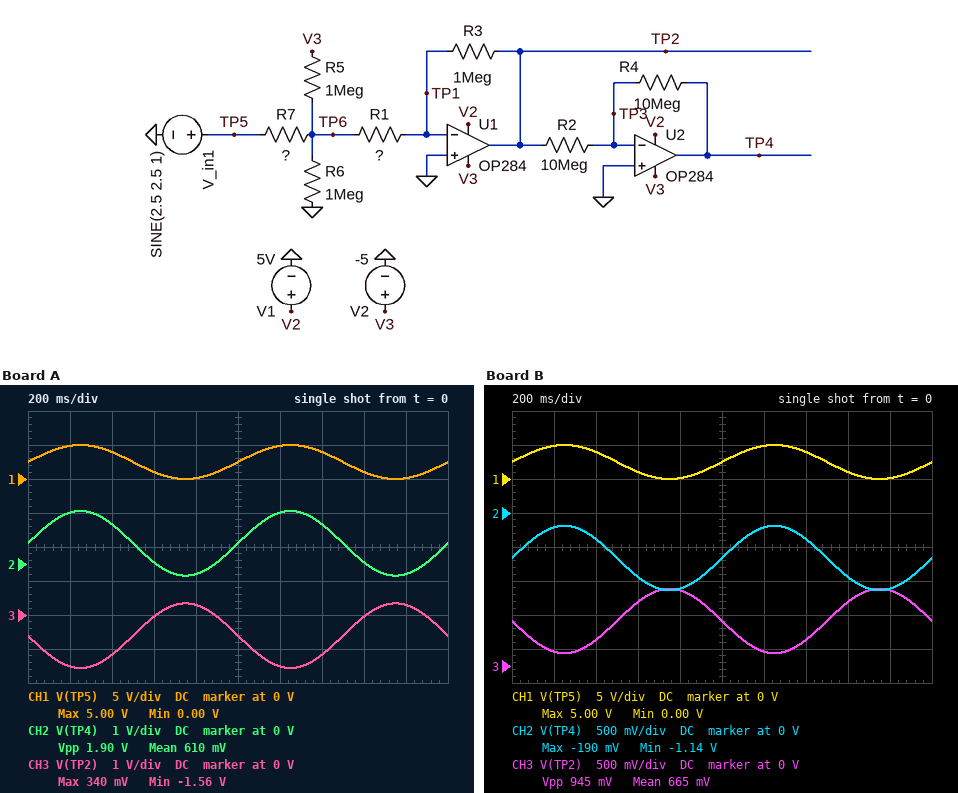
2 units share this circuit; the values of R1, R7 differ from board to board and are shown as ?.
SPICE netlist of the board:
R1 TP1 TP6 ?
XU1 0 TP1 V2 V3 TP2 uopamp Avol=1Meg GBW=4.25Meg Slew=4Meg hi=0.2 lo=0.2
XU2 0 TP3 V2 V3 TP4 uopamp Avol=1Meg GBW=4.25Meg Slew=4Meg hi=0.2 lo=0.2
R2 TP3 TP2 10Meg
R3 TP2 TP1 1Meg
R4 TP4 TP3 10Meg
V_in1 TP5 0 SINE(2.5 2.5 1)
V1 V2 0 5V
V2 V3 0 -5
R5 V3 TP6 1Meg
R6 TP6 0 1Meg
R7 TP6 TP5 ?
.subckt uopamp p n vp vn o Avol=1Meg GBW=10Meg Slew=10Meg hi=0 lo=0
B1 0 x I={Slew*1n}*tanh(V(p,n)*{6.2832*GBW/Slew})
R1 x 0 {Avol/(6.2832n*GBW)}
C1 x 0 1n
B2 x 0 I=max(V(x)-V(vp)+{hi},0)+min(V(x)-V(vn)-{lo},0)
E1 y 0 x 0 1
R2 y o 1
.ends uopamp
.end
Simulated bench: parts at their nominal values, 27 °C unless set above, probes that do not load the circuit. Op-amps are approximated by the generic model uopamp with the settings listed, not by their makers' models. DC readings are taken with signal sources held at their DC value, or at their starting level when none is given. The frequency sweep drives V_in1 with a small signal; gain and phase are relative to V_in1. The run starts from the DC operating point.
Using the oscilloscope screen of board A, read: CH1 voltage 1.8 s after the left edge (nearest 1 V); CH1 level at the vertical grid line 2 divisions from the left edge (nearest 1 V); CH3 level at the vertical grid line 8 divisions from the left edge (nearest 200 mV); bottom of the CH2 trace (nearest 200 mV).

0 V
4 V
0 V
-400 mV
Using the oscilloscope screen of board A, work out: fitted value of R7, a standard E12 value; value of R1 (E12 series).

180 kΩ
1.8 MΩ
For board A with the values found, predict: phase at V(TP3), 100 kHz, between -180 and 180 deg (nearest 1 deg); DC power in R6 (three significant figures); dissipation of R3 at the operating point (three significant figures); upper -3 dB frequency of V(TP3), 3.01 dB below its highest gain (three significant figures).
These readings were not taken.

-95 deg
1.20 µW
371 nW
5.93 MHz
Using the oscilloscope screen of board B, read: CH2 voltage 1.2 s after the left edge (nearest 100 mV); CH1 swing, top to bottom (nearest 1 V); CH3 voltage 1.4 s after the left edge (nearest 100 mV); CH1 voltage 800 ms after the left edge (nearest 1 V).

-200 mV
5 V
400 mV
0 V
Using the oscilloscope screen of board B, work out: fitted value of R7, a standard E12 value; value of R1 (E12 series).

1.2 MΩ
1.2 MΩ
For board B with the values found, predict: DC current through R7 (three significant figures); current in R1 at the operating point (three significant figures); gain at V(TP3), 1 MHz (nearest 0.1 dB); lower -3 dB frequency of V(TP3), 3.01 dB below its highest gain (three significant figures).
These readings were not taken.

2.75 µA
663 nA
-28.5 dB
968 kHz
